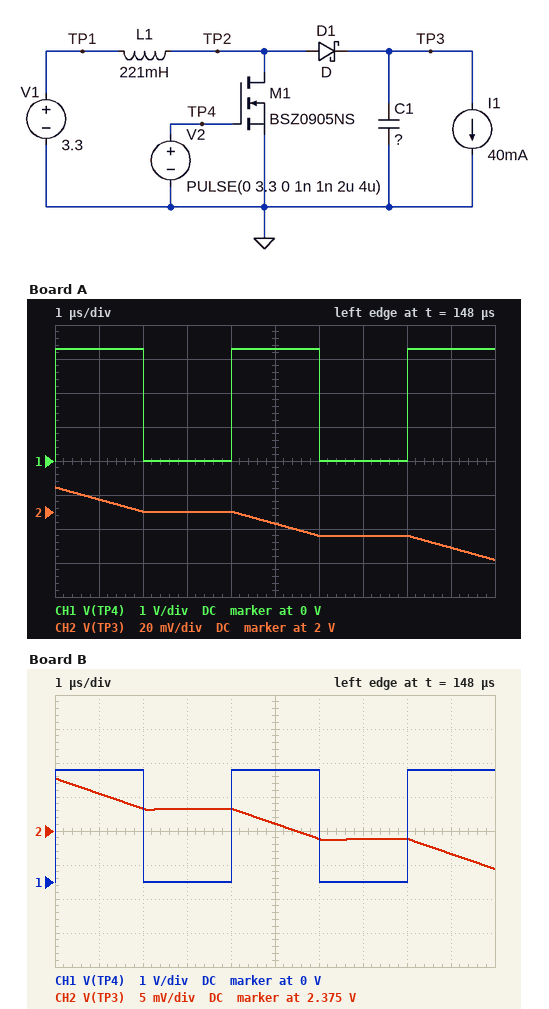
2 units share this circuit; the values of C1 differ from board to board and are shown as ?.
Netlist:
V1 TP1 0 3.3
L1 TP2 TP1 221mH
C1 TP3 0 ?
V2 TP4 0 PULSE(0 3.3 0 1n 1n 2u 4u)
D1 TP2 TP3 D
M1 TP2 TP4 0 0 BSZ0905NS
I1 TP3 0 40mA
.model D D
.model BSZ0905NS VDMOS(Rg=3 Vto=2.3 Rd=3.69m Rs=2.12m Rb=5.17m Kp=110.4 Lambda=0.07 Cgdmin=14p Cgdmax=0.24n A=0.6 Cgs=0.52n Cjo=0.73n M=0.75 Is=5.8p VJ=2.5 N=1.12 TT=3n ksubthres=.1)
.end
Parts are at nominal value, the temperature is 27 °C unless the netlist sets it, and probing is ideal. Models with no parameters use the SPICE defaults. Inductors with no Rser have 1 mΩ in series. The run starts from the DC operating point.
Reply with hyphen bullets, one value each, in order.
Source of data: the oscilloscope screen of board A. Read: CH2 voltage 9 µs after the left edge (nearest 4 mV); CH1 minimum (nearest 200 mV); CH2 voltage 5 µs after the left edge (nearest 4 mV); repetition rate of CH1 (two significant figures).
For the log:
- 1.980 V
- 0 V
- 1.992 V
- 250 kHz
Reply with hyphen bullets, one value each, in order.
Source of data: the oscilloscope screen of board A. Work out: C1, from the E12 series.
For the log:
- 5.6 µF
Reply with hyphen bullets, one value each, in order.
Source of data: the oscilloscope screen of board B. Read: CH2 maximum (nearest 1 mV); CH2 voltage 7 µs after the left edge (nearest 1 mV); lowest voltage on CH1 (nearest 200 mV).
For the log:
- 2.383 V
- 2.374 V
- 0 V
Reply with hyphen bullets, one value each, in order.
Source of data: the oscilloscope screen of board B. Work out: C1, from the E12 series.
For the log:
- 18 µF
